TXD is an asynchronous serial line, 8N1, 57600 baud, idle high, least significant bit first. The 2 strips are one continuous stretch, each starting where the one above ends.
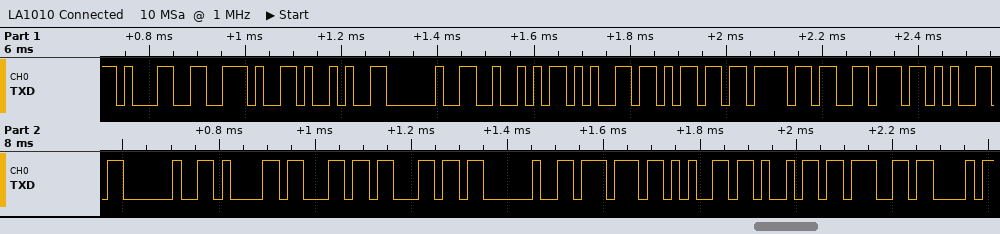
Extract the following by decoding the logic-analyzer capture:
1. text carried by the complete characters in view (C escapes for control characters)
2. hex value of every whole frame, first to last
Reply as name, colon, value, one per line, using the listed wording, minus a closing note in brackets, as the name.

text carried by the complete characters in view: "1.) Remove all weig"
hex value of every whole frame, first to last: 31 2E 29 20 52 65 6D 6F 76 65 20 61 6C 6C 20 77 65 69 67
